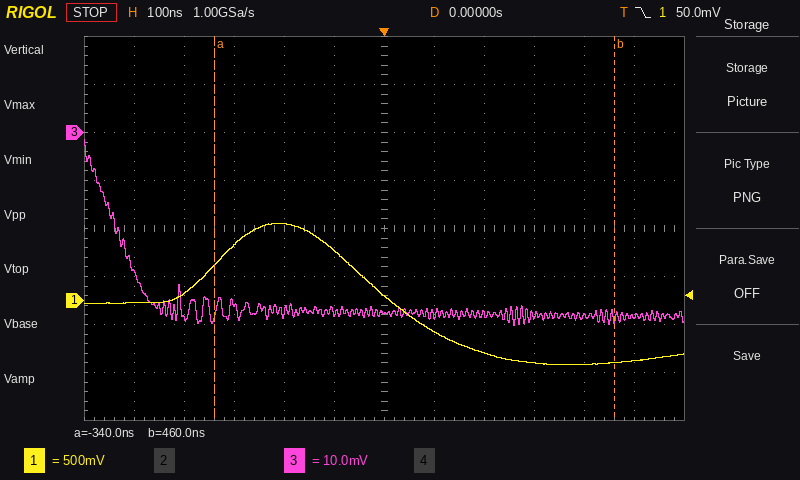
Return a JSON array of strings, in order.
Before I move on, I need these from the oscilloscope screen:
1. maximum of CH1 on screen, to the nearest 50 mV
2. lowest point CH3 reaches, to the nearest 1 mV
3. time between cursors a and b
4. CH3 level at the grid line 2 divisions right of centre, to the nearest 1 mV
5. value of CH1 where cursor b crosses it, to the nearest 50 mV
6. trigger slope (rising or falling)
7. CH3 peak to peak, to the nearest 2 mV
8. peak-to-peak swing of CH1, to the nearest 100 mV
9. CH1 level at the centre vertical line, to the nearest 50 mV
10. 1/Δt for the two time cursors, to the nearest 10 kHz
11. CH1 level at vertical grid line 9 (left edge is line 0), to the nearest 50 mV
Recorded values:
["800 mV", "-40 mV", "800 ns", "-38 mV", "-650 mV", "falling", "38 mV", "1.50 V", "50 mV", "1.25 MHz", "-650 mV"]
